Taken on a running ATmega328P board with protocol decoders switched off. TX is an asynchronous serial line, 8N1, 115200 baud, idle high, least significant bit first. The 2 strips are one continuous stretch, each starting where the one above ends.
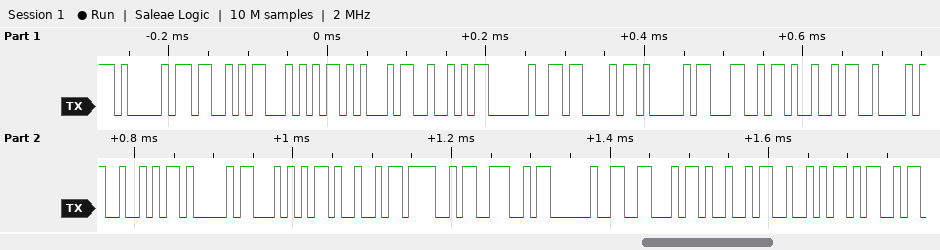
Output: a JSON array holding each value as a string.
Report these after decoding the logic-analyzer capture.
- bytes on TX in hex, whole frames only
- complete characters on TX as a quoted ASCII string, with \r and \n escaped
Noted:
["41 53 54 45 52 20 43 41 4C 49 42 52 41 54 49 4F 4E 20 46 49 52 4D", "\"ASTER CALIBRATION FIRM\""]
